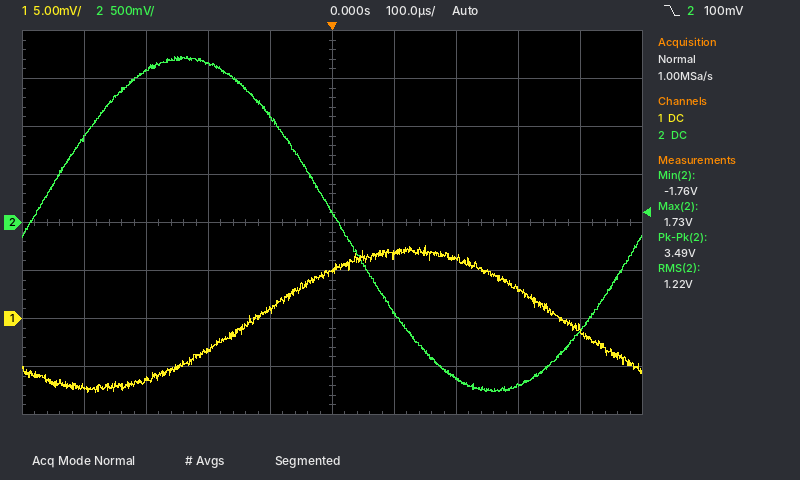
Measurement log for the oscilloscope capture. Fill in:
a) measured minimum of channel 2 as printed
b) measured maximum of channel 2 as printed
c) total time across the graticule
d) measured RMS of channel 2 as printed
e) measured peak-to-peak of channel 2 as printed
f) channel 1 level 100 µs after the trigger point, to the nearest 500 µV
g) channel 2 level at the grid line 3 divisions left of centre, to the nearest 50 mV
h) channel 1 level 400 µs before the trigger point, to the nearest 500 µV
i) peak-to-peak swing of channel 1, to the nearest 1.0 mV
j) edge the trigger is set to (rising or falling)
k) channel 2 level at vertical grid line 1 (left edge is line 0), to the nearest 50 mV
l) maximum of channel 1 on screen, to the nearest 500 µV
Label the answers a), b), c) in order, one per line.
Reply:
a) -1.76 V
b) 1.73 V
c) 1 ms
d) 1.22 V
e) 3.49 V
f) 6.5 mV
g) 1.60 V
h) -7.0 mV
i) 15.0 mV
j) falling
k) 900 mV
l) 7.5 mV
